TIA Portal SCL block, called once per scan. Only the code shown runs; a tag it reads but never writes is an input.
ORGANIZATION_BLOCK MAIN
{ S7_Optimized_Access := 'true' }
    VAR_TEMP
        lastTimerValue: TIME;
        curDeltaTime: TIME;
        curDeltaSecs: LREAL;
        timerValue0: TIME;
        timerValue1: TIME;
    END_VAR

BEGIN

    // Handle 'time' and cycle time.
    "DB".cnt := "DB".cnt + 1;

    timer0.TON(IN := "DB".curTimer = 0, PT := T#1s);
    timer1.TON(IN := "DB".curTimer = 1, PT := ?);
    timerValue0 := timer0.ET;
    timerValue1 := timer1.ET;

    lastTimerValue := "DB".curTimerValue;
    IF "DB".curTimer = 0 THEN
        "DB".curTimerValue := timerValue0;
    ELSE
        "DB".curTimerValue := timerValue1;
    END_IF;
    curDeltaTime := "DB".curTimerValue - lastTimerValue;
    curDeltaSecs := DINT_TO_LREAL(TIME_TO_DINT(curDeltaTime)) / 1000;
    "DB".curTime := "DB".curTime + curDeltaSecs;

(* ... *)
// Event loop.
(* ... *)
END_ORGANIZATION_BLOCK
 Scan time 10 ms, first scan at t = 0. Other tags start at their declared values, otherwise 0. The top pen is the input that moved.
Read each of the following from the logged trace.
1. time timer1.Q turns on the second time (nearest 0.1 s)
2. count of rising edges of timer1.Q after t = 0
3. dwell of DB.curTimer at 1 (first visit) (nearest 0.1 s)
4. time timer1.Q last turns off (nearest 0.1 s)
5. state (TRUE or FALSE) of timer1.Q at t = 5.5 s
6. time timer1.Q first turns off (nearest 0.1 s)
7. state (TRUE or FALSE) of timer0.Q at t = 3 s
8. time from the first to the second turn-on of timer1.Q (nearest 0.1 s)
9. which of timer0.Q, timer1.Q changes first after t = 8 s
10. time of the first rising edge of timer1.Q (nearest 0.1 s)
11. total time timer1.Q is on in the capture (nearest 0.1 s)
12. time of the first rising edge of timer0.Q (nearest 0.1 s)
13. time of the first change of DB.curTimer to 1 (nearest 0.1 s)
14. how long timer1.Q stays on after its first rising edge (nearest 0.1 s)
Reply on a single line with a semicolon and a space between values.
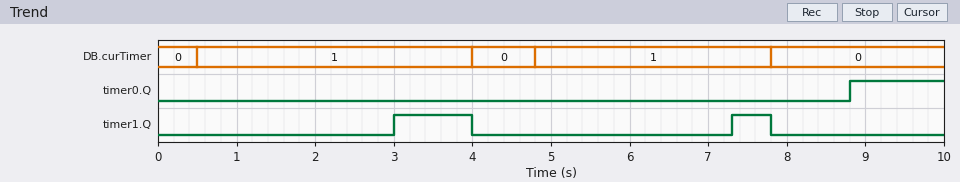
7.3 s; 2; 3.5 s; 7.8 s; FALSE; 4.0 s; FALSE; 4.3 s; timer0.Q; 3.0 s; 1.5 s; 8.8 s; 0.5 s; 1.0 s
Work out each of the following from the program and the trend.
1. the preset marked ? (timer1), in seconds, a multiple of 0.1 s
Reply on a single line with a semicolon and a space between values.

2.5 s
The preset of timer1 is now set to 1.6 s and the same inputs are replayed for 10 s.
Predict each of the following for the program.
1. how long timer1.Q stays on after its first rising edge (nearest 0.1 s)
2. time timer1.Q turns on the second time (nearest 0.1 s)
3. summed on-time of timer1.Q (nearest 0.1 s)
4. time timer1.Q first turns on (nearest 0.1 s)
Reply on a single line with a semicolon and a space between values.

1.9 s; 6.4 s; 3.3 s; 2.1 s
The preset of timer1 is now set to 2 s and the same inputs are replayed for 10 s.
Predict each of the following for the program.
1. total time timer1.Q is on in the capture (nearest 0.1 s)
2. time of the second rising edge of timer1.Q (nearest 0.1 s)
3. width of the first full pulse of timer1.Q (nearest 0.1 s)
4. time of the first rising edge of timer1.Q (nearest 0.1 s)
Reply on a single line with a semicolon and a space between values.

2.5 s; 6.8 s; 1.5 s; 2.5 s
